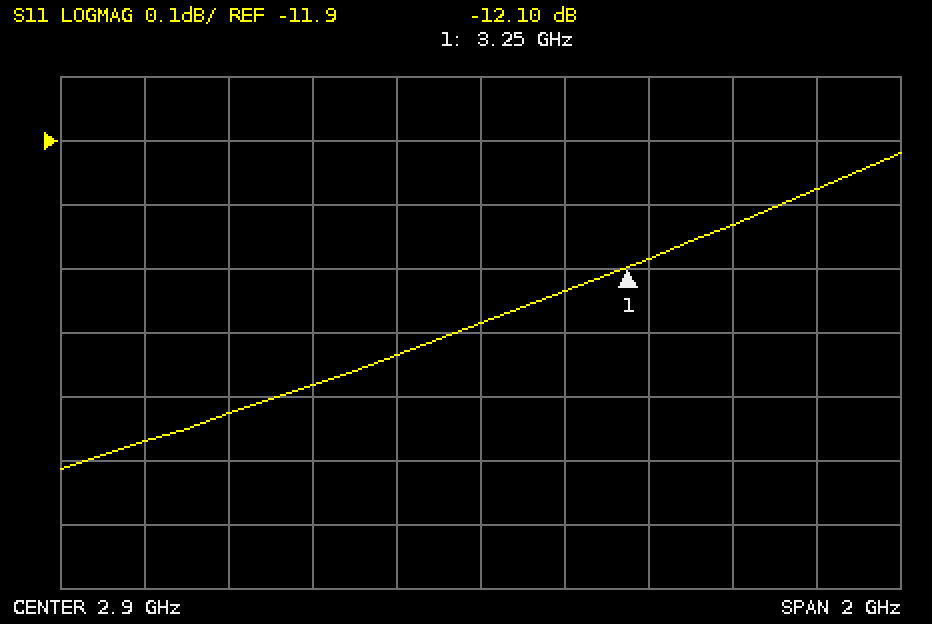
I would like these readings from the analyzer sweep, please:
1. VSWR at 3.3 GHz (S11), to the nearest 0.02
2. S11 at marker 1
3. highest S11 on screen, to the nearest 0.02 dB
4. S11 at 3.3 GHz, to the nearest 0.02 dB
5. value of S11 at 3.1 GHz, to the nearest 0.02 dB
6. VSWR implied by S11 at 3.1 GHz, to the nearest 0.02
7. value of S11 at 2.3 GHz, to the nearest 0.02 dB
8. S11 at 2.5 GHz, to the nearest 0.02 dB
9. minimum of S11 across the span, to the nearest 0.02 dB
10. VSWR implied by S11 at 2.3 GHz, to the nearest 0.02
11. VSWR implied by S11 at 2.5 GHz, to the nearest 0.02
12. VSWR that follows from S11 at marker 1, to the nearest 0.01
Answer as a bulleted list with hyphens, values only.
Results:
- 1.66
- -12.10 dB
- -11.92 dB
- -12.08 dB
- -12.14 dB
- 1.66
- -12.32 dB
- -12.28 dB
- -12.42 dB
- 1.64
- 1.64
- 1.66
